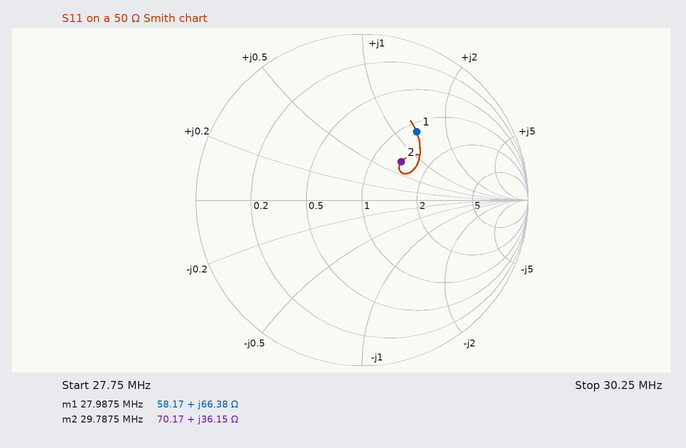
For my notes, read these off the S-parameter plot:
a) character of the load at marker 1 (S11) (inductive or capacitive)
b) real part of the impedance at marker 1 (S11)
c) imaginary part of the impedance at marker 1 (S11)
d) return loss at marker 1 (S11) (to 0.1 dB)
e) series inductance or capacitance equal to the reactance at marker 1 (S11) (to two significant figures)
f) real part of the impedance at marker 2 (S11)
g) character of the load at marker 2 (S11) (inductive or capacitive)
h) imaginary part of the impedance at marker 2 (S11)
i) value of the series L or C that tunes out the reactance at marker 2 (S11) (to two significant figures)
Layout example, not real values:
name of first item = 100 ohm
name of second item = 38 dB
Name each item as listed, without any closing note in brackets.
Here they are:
character of the load at marker 1 (S11) = inductive
real part of the impedance at marker 1 = 58.17 Ω
imaginary part of the impedance at marker 1 = +66.38 Ω
return loss at marker 1 (S11) = 5.6 dB
series inductance or capacitance equal to the reactance at marker 1 (S11) = 380 nH
real part of the impedance at marker 2 = 70.17 Ω
character of the load at marker 2 (S11) = inductive
imaginary part of the impedance at marker 2 = +36.15 Ω
value of the series L or C that tunes out the reactance at marker 2 (S11) = 150 pF
